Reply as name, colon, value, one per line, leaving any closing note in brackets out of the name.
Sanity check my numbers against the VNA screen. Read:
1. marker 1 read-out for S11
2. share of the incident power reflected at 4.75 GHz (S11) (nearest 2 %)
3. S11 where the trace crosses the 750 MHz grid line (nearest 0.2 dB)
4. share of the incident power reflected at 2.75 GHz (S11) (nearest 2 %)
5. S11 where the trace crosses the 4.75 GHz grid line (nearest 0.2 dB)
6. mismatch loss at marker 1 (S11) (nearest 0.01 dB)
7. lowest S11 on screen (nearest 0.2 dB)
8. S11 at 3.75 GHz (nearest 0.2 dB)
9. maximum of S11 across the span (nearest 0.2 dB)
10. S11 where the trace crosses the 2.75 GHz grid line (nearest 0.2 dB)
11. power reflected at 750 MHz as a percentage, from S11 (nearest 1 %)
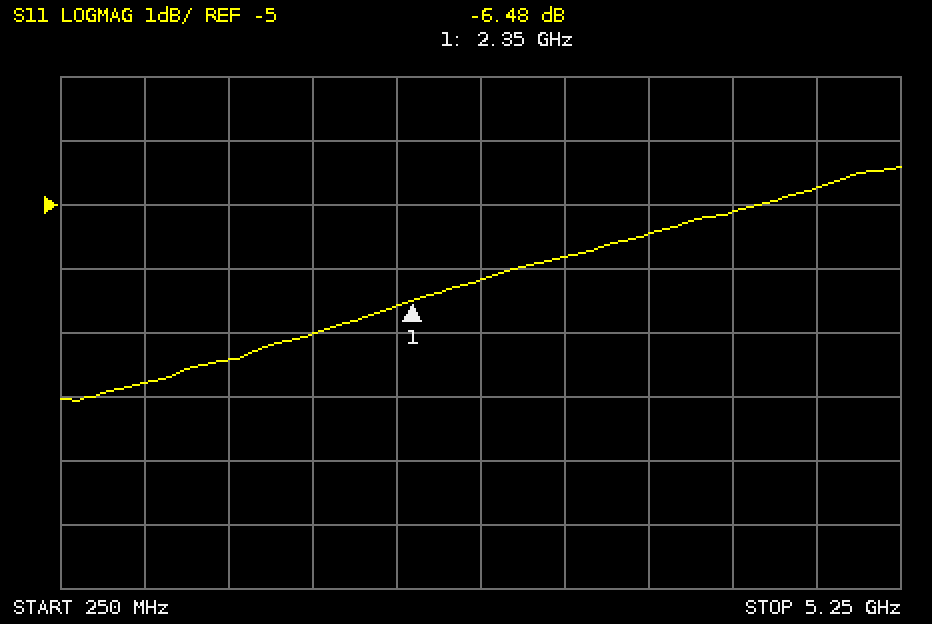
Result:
marker 1 read-out for S11: -6.48 dB
share of the incident power reflected at 4.75 GHz (S11): 34 %
S11 where the trace crosses the 750 MHz grid line: -7.8 dB
share of the incident power reflected at 2.75 GHz (S11): 24 %
S11 where the trace crosses the 4.75 GHz grid line: -4.8 dB
mismatch loss at marker 1 (S11): 1.11 dB
lowest S11 on screen: -8.0 dB
S11 at 3.75 GHz: -5.4 dB
maximum of S11 across the span: -4.4 dB
S11 where the trace crosses the 2.75 GHz grid line: -6.2 dB
power reflected at 750 MHz as a percentage, from S11: 17 %
